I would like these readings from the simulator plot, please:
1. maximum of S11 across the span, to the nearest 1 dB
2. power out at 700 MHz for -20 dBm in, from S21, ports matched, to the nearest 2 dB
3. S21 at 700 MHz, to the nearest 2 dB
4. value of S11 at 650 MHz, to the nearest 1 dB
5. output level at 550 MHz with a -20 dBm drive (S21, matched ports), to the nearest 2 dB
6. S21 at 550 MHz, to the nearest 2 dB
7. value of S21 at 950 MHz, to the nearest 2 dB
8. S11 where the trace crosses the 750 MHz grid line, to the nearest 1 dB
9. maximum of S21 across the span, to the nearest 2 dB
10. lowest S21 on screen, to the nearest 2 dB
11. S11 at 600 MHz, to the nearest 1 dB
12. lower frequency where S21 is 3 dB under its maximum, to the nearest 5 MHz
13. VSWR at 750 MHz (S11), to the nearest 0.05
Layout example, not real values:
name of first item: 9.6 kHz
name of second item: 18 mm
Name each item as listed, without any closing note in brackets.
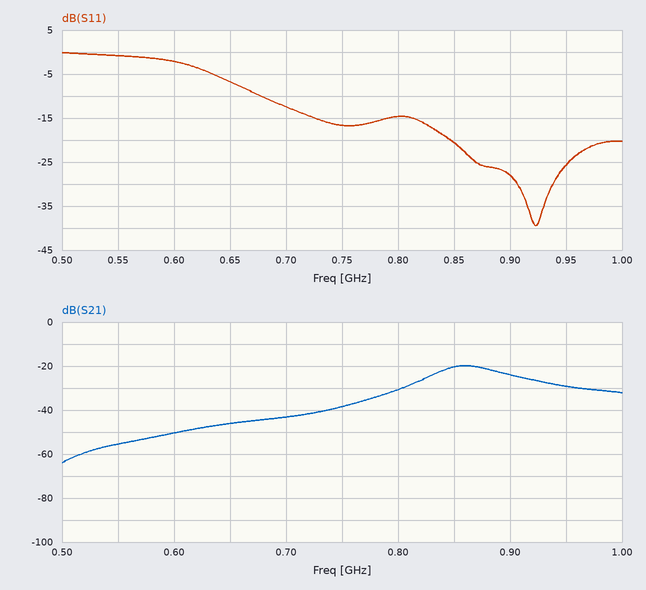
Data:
maximum of S11 across the span, to the nearest 1 dB: 0 dB
power out at 700 MHz for -20 dBm in, from S21, ports matched, to the nearest 2 dB: -64 dBm
S21 at 700 MHz, to the nearest 2 dB: -44 dB
value of S11 at 650 MHz, to the nearest 1 dB: -7 dB
output level at 550 MHz with a -20 dBm drive (S21, matched ports), to the nearest 2 dB: -76 dBm
S21 at 550 MHz, to the nearest 2 dB: -56 dB
value of S21 at 950 MHz, to the nearest 2 dB: -30 dB
S11 where the trace crosses the 750 MHz grid line, to the nearest 1 dB: -17 dB
maximum of S21 across the span, to the nearest 2 dB: -20 dB
lowest S21 on screen, to the nearest 2 dB: -64 dB
S11 at 600 MHz, to the nearest 1 dB: -2 dB
lower frequency where S21 is 3 dB under its maximum, to the nearest 5 MHz: 835 MHz
VSWR at 750 MHz (S11), to the nearest 0.05: 1.35
